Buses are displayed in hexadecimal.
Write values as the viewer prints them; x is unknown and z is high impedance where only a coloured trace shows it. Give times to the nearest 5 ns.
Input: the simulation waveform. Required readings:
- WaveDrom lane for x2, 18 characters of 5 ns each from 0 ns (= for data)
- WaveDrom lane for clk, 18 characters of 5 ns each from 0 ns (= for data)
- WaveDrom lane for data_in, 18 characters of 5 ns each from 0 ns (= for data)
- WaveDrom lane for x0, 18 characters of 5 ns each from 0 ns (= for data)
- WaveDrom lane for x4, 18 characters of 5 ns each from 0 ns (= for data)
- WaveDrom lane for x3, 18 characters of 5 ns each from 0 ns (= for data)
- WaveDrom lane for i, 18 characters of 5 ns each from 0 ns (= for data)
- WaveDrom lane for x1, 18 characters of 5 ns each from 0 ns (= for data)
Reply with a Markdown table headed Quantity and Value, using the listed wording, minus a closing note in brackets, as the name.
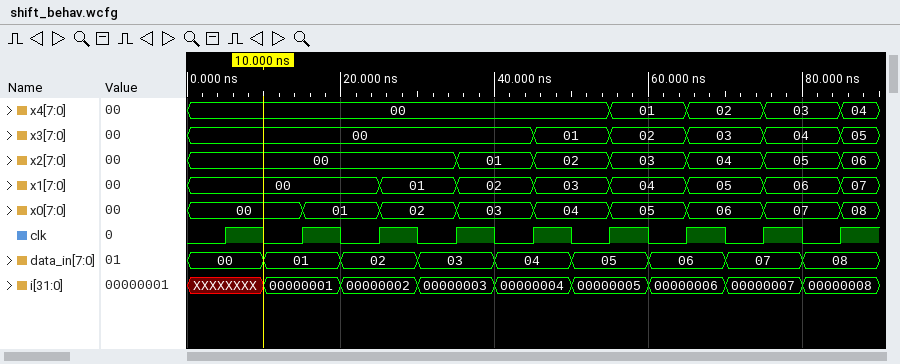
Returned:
| Quantity | Value |
|---|---|
| WaveDrom lane for x2, 18 characters of 5 ns each from 0 ns | {name: 'x2', wave: '=......=.=.=.=.=.=', data: '00 01 02 03 04 05 06'} |
| WaveDrom lane for clk, 18 characters of 5 ns each from 0 ns | {name: 'clk', wave: '010101010101010101'} |
| WaveDrom lane for data_in, 18 characters of 5 ns each from 0 ns | {name: 'data_in', wave: '=.=.=.=.=.=.=.=.=.', data: '00 01 02 03 04 05 06 07 08'} |
| WaveDrom lane for x0, 18 characters of 5 ns each from 0 ns | {name: 'x0', wave: '=..=.=.=.=.=.=.=.=', data: '00 01 02 03 04 05 06 07 08'} |
| WaveDrom lane for x4, 18 characters of 5 ns each from 0 ns | {name: 'x4', wave: '=..........=.=.=.=', data: '00 01 02 03 04'} |
| WaveDrom lane for x3, 18 characters of 5 ns each from 0 ns | {name: 'x3', wave: '=........=.=.=.=.=', data: '00 01 02 03 04 05'} |
| WaveDrom lane for i, 18 characters of 5 ns each from 0 ns | {name: 'i', wave: 'x.=.=.=.=.=.=.=.=.', data: '00000001 00000002 00000003 00000004 00000005 00000006 00000007 00000008'} |
| WaveDrom lane for x1, 18 characters of 5 ns each from 0 ns | {name: 'x1', wave: '=....=.=.=.=.=.=.=', data: '00 01 02 03 04 05 06 07'} |
